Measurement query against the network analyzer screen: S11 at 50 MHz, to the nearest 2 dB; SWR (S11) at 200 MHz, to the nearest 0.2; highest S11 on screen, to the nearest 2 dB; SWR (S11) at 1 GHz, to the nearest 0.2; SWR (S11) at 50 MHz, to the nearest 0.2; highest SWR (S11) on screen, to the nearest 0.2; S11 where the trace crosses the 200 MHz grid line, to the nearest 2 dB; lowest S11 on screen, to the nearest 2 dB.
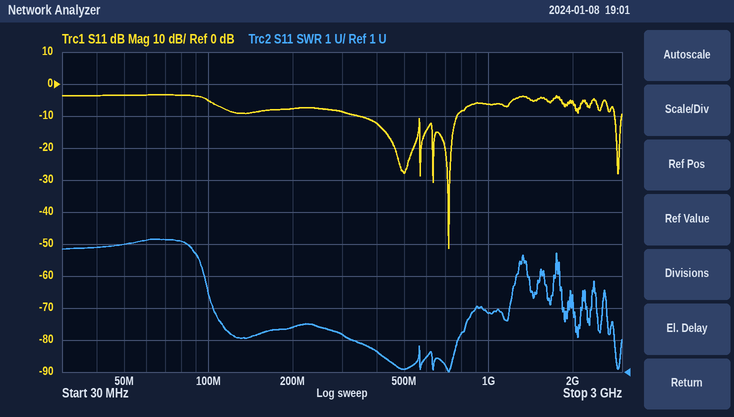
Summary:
-4 dB
2.4
-4 dB
2.8
5.0
5.2
-8 dB
-52 dB
